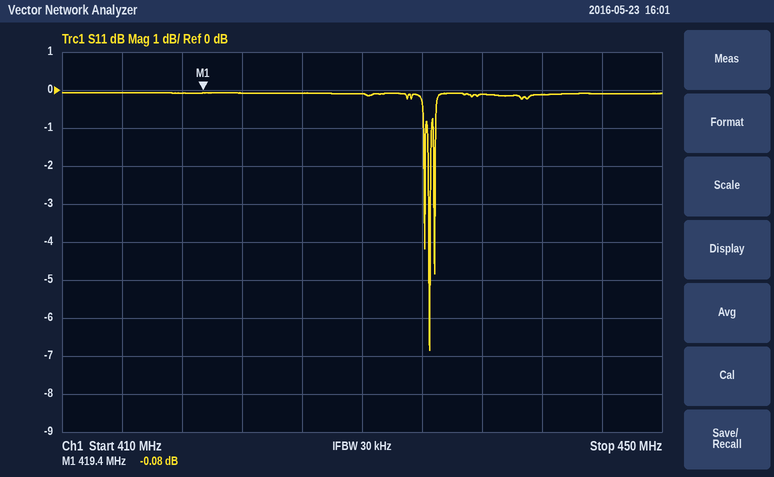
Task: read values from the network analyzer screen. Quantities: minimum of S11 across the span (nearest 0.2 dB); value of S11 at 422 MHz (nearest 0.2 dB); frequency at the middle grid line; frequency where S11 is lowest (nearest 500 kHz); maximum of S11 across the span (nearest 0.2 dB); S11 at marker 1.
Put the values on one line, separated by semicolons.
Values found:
-6.8 dB; 0.0 dB; 430 MHz; 434.5 MHz; 0.0 dB; -0.08 dB
